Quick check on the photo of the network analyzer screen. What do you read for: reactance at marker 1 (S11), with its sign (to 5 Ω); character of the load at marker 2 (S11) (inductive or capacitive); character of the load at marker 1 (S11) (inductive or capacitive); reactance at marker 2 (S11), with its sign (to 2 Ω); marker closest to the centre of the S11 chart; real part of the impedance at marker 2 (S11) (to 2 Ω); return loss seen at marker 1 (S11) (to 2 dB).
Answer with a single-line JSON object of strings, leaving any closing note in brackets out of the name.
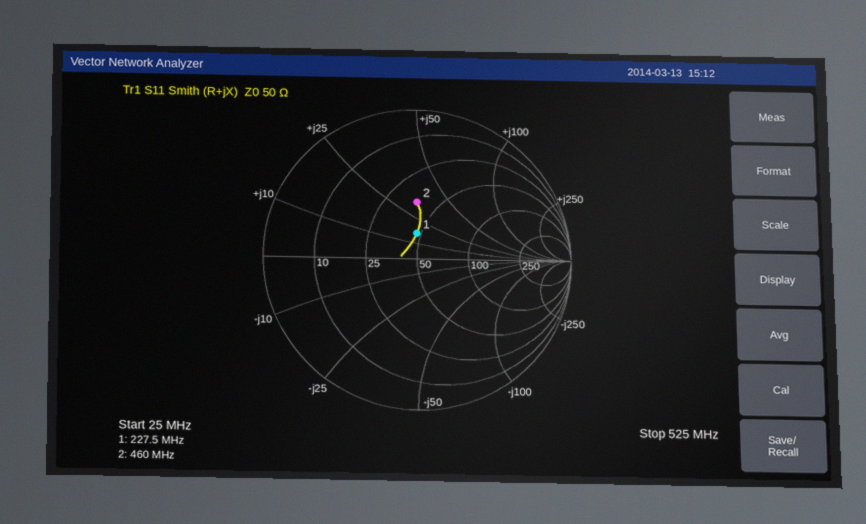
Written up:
{"reactance at marker 1 (S11), with its sign": "+15 Ω", "character of the load at marker 2 (S11)": "inductive", "character of the load at marker 1 (S11)": "inductive", "reactance at marker 2 (S11), with its sign": "+34 Ω", "marker closest to the centre of the S11 chart": "marker 1", "real part of the impedance at marker 2 (S11)": "38 Ω", "return loss seen at marker 1 (S11)": "16 dB"}
